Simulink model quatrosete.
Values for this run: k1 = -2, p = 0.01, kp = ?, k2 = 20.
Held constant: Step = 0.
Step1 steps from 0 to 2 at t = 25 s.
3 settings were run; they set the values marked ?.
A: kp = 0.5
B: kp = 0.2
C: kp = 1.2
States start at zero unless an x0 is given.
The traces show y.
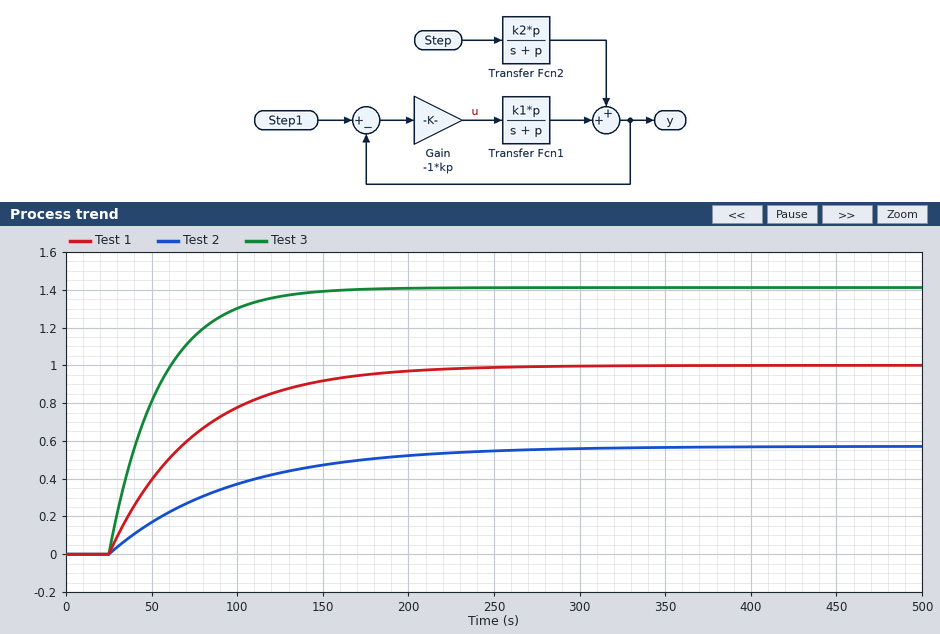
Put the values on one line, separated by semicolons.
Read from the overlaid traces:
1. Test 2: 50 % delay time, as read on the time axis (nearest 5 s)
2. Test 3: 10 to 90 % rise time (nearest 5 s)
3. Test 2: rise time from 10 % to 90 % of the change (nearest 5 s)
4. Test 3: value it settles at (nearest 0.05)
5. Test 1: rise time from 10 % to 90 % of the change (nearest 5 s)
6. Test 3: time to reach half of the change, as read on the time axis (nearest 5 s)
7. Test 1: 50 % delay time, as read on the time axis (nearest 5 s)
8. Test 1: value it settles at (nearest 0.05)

75 s; 65 s; 155 s; 1.40; 110 s; 45 s; 60 s; 1.00
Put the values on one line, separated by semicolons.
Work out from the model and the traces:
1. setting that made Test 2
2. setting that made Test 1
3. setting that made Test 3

B; A; C
